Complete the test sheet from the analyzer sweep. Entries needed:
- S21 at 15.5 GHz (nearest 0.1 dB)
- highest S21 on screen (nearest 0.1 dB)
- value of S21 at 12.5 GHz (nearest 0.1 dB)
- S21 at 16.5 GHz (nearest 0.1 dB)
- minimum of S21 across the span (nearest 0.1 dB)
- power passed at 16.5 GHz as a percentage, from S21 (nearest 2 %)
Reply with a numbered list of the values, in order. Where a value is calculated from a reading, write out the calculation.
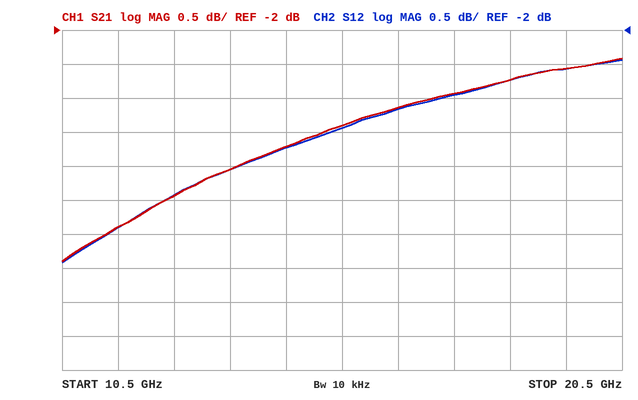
1. -3.4 dB
2. -2.4 dB
3. -4.4 dB
4. -3.1 dB
5. -5.4 dB
6. 10^(-3.1/10) ≈ 49.0 %, so 48 % to the nearest 2 %
